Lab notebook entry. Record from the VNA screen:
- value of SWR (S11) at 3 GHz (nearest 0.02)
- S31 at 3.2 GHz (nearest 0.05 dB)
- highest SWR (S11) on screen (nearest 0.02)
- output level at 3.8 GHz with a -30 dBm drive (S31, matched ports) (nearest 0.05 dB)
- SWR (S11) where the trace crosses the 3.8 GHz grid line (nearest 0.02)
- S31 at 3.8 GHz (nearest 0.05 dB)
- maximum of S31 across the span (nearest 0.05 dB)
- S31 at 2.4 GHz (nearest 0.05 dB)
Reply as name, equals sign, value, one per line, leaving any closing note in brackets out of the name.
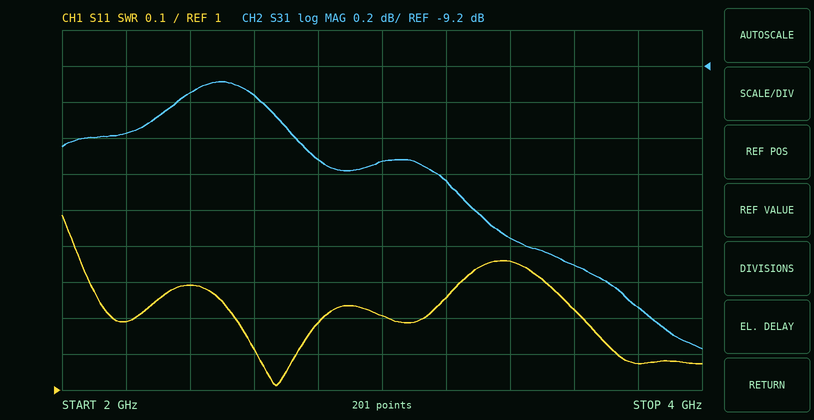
value of SWR (S11) at 3 GHz = 1.20
S31 at 3.2 GHz = -9.85 dB
highest SWR (S11) on screen = 1.48
output level at 3.8 GHz with a -30 dBm drive (S31, matched ports) = -40.55 dBm
SWR (S11) where the trace crosses the 3.8 GHz grid line = 1.08
S31 at 3.8 GHz = -10.55 dB
maximum of S31 across the span = -9.30 dB
S31 at 2.4 GHz = -9.35 dB
